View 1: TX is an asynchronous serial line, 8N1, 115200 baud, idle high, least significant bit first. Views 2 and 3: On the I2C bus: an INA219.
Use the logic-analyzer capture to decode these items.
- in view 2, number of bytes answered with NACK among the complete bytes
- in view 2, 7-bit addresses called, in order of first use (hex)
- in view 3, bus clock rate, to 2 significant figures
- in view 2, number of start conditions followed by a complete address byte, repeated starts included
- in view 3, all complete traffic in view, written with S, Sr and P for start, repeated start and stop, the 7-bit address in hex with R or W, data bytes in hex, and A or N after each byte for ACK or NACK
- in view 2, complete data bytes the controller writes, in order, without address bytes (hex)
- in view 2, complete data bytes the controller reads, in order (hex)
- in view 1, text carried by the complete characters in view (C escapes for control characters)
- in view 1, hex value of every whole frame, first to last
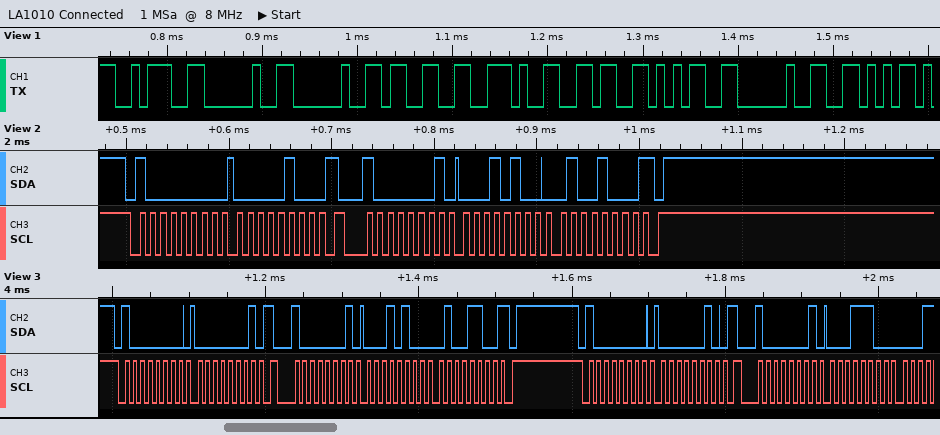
1
0x40
100 kHz
2
S 40W A 01 A Sr 40R A 14 A 4C N P S 40W A 02 A Sr 40R A 1C A
04
14 48
":  3.65 V"
3A 20 20 33 2E 36 35 20 56
